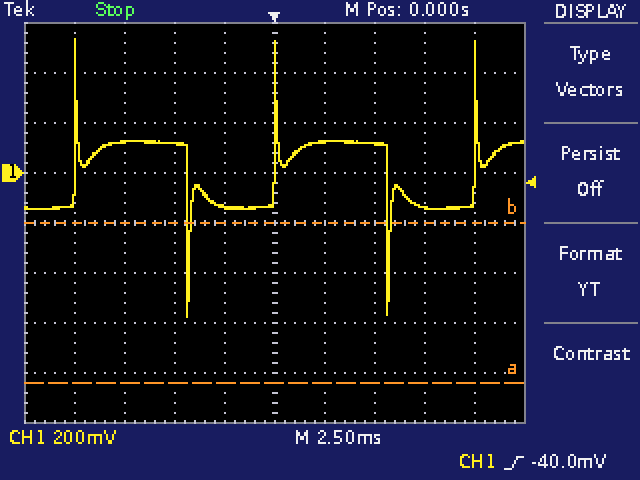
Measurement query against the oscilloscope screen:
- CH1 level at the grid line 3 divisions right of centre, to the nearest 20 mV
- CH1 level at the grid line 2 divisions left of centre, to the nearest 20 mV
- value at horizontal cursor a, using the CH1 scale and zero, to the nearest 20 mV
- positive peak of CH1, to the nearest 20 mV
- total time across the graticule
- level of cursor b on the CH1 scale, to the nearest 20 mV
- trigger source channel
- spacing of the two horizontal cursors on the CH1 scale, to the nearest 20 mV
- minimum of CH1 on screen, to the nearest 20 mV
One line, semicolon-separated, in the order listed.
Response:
-140 mV; 120 mV; -840 mV; 540 mV; 25 ms; -200 mV; CH1; 640 mV; -580 mV
